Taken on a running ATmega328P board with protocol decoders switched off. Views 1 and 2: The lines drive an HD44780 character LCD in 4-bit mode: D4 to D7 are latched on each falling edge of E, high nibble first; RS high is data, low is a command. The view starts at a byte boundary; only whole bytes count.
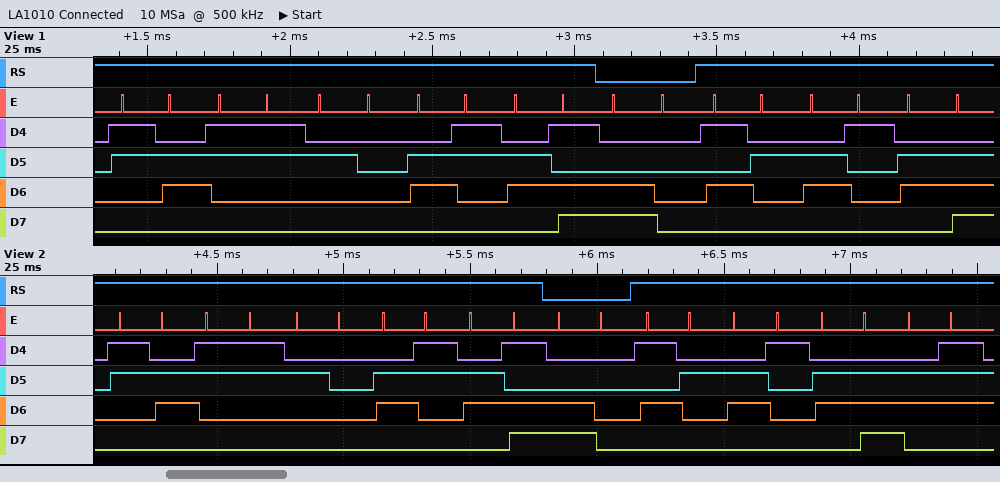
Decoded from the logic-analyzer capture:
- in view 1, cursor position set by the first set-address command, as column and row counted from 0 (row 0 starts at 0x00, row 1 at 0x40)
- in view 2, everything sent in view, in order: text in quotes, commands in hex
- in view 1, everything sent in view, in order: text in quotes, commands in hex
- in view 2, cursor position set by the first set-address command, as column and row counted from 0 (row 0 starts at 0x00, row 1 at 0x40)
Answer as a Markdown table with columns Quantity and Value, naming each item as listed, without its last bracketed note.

| Quantity | Value |
|---|---|
| in view 1, cursor position set by the first set-address command, as column and row counted from 0 | column 0, row 1 |
| in view 2, everything sent in view, in order: text in quotes, commands in hex | "63 cm" 0xC0 "Rang" |
| in view 1, everything sent in view, in order: text in quotes, commands in hex | "63 cm" 0xC0 "Ran" |
| in view 2, cursor position set by the first set-address command, as column and row counted from 0 | column 0, row 1 |
